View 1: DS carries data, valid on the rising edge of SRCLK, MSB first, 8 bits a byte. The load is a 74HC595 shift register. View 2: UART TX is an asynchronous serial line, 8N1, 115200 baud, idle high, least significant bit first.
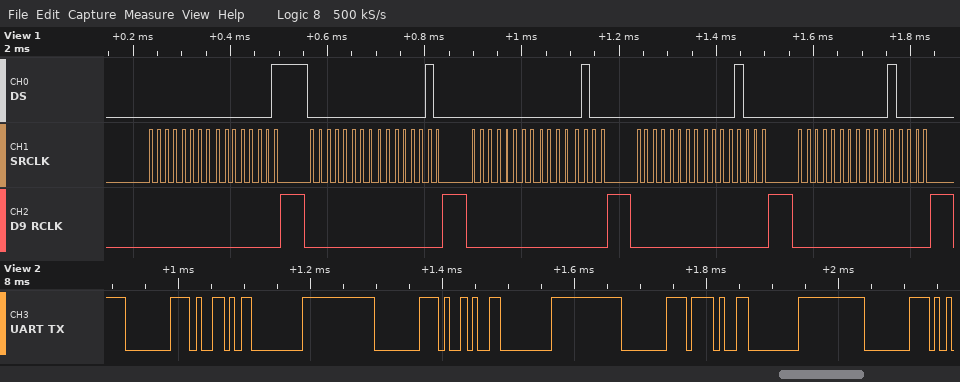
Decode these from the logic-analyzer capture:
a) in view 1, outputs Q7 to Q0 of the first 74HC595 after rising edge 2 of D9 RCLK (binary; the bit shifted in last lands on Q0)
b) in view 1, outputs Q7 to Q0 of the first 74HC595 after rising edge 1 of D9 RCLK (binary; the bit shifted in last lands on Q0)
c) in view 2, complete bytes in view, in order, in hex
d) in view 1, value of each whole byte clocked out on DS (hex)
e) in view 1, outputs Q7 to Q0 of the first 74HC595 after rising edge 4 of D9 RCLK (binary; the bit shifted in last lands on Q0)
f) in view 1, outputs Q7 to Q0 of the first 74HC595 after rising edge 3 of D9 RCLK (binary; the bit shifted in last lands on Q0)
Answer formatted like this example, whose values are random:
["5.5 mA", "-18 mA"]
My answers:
["00000010", "00000001", "80 59 00 80 29 00 80 2F 00 80", "0x00 0x01 0x00 0x02 0x00 0x04 0x00 0x08 0x00 0x10", "00001000", "00000100"]
